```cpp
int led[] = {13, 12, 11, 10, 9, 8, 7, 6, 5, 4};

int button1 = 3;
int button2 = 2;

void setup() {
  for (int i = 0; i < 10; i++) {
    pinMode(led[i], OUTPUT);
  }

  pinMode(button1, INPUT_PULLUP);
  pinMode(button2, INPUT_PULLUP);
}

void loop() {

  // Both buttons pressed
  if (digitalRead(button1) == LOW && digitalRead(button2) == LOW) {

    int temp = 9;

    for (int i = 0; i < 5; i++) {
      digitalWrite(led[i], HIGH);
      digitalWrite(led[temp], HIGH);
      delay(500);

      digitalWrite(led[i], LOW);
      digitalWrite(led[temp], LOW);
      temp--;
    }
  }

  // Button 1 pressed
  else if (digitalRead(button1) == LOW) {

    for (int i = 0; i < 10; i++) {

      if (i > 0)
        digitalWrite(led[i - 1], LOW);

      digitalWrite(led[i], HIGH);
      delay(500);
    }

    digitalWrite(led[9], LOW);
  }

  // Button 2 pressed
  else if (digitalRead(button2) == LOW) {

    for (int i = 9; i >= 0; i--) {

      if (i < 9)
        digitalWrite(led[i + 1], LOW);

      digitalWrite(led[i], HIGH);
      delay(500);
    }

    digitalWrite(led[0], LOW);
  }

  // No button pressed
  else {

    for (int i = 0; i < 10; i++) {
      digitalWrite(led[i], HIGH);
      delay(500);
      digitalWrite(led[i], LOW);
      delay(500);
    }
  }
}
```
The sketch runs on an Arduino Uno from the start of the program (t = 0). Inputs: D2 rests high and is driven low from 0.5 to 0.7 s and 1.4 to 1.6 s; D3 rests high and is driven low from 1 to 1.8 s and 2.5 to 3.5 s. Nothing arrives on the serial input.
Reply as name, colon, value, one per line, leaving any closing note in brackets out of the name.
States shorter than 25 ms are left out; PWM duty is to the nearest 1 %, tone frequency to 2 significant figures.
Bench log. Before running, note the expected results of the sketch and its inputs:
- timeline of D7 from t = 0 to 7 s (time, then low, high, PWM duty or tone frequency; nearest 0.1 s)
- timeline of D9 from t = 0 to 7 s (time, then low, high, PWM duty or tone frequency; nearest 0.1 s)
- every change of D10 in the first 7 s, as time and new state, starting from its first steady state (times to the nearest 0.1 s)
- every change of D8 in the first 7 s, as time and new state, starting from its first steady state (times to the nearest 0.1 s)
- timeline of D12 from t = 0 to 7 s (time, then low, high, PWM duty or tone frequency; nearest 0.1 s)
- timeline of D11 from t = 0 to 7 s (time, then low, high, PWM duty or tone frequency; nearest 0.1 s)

timeline of D7 from t = 0 to 7 s: 0 s low; 6 s high; 6.5 s low
timeline of D9 from t = 0 to 7 s: 0 s low; 4 s high; 4.5 s low
every change of D10 in the first 7 s, as time and new state, starting from its first steady state: 0 s low; 3 s high; 3.5 s low
every change of D8 in the first 7 s, as time and new state, starting from its first steady state: 0 s low; 5 s high; 5.5 s low
timeline of D12 from t = 0 to 7 s: 0 s low; 1 s high; 1.5 s low
timeline of D11 from t = 0 to 7 s: 0 s low; 2 s high; 2.5 s low
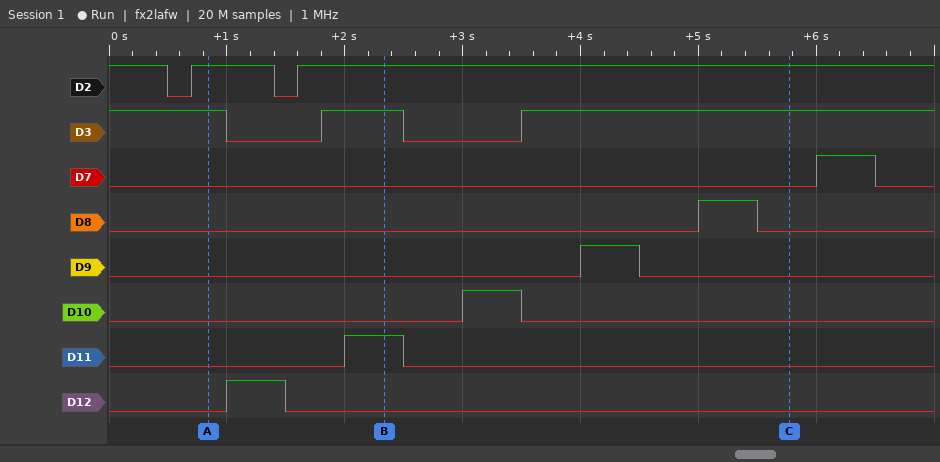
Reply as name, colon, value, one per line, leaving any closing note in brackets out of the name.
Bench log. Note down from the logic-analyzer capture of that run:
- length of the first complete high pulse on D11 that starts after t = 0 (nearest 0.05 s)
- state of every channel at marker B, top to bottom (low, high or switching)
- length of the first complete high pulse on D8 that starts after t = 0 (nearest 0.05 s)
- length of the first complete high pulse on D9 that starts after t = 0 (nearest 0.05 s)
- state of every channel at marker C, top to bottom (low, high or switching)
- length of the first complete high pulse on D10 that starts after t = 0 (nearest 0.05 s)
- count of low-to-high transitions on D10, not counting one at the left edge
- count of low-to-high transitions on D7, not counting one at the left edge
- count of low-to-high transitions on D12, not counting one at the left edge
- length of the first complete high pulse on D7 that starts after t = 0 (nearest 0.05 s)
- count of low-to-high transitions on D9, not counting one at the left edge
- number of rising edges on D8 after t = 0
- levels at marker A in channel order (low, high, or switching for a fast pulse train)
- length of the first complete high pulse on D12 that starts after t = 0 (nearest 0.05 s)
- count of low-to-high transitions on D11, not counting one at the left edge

length of the first complete high pulse on D11 that starts after t = 0: 0.50 s
state of every channel at marker B, top to bottom: D2 high, D3 high, D7 low, D8 low, D9 low, D10 low, D11 high, D12 low
length of the first complete high pulse on D8 that starts after t = 0: 0.50 s
length of the first complete high pulse on D9 that starts after t = 0: 0.50 s
state of every channel at marker C, top to bottom: D2 high, D3 high, D7 low, D8 low, D9 low, D10 low, D11 low, D12 low
length of the first complete high pulse on D10 that starts after t = 0: 0.50 s
count of low-to-high transitions on D10, not counting one at the left edge: 1
count of low-to-high transitions on D7, not counting one at the left edge: 1
count of low-to-high transitions on D12, not counting one at the left edge: 1
length of the first complete high pulse on D7 that starts after t = 0: 0.50 s
count of low-to-high transitions on D9, not counting one at the left edge: 1
number of rising edges on D8 after t = 0: 1
levels at marker A in channel order: D2 high, D3 high, D7 low, D8 low, D9 low, D10 low, D11 low, D12 low
length of the first complete high pulse on D12 that starts after t = 0: 0.50 s
count of low-to-high transitions on D11, not counting one at the left edge: 1
